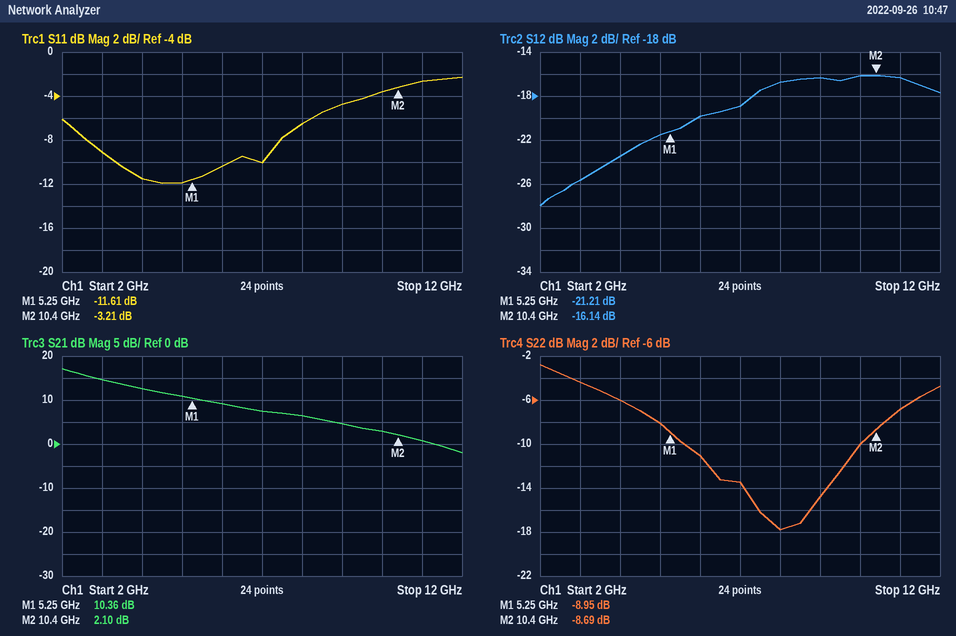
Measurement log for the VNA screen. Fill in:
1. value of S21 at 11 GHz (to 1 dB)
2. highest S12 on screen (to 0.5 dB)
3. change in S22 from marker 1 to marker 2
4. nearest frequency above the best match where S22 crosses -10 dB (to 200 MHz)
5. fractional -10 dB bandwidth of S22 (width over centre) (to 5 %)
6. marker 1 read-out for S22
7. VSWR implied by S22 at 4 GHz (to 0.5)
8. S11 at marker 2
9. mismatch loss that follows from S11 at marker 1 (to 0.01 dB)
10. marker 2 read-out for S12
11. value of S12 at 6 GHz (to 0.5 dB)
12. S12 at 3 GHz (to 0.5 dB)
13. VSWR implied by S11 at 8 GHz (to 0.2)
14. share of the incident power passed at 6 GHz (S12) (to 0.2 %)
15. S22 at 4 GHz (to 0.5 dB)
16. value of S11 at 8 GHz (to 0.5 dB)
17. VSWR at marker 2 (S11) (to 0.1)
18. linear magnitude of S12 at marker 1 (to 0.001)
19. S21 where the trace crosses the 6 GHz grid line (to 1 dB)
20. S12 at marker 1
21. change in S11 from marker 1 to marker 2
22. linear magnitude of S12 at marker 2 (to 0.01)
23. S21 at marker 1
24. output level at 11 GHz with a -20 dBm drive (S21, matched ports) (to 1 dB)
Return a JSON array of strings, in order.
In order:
["1 dB", "-16.0 dB", "0.26 dB", "10.0 GHz", "55 %", "-8.95 dB", "3.0", "-3.21 dB", "0.31 dB", "-16.14 dB", "-20.0 dB", "-25.5 dB", "2.8", "1.0 %", "-6.0 dB", "-6.5 dB", "5.5", "0.087", "9 dB", "-21.21 dB", "8.40 dB", "0.16", "10.36 dB", "-19 dBm"]
